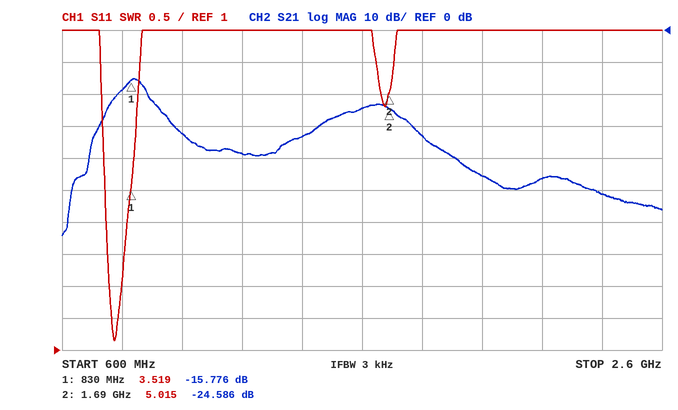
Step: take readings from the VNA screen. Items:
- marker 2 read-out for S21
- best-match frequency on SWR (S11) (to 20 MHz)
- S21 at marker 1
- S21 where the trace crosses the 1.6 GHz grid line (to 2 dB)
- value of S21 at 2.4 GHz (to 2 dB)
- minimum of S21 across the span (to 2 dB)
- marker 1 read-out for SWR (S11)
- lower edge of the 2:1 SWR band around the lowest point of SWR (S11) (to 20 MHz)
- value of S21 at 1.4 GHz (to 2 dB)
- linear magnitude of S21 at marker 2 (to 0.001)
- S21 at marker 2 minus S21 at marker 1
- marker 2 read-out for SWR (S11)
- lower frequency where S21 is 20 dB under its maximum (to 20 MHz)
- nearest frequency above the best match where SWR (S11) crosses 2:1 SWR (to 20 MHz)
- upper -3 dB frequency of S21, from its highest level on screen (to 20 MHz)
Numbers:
-24.586 dB
780 MHz
-15.776 dB
-24 dB
-52 dB
-64 dB
3.519
760 MHz
-34 dB
0.059
-8.810 dB
5.015
700 MHz
800 MHz
880 MHz
